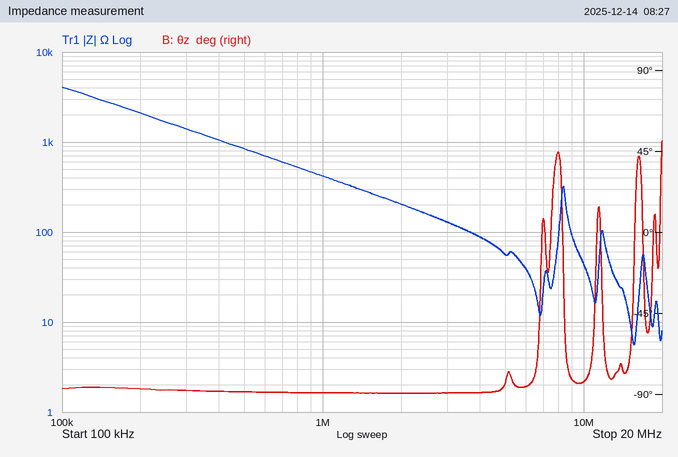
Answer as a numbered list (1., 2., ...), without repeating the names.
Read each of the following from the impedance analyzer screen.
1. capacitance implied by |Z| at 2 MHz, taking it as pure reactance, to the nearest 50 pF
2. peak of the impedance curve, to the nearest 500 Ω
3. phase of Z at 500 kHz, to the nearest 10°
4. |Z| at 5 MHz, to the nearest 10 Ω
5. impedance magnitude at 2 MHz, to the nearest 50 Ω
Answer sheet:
1. 400 pF
2. 4.0 kΩ
3. -90°
4. 60 Ω
5. 200 Ω
